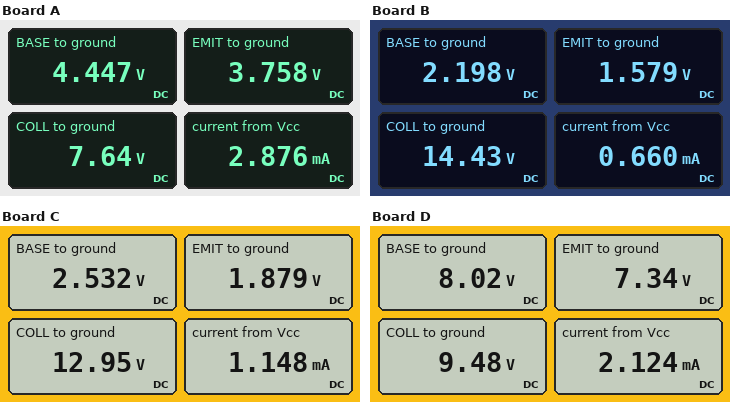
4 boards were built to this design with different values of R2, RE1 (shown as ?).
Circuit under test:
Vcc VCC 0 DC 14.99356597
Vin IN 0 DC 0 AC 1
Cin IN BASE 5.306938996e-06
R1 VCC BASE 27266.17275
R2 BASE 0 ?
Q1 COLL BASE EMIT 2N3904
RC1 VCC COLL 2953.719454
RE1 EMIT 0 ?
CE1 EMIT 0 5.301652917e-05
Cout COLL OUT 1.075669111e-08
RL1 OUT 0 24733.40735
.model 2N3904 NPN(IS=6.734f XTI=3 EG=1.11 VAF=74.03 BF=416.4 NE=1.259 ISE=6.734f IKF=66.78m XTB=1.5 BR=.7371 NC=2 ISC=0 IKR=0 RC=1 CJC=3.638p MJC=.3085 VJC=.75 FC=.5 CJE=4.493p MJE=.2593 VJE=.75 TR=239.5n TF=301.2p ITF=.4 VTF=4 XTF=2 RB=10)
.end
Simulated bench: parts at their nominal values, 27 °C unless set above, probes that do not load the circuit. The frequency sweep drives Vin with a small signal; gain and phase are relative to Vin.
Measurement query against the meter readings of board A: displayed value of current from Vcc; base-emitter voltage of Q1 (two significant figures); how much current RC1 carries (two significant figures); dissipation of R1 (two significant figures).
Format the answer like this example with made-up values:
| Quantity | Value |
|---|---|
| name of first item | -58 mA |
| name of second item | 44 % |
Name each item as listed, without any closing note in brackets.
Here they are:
| Quantity | Value |
|---|---|
| displayed value of current from Vcc | 2.876 mA |
| base-emitter voltage of Q1 | 690 mV |
| how much current RC1 carries | 2.5 mA |
| dissipation of R1 | 4.1 mW |
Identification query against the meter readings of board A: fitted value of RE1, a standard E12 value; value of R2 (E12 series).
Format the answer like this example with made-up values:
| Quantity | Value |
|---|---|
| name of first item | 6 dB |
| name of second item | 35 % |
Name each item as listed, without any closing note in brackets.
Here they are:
| Quantity | Value |
|---|---|
| fitted value of RE1, a standard E12 value | 1.5 kΩ |
| value of R2 | 12 kΩ |
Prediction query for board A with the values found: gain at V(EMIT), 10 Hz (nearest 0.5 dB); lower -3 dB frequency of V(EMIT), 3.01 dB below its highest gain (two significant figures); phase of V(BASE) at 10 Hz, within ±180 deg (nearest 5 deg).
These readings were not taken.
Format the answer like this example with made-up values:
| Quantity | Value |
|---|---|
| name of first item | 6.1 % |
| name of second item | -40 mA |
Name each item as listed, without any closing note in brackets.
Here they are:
| Quantity | Value |
|---|---|
| gain at V(EMIT), 10 Hz | -1.0 dB |
| lower -3 dB frequency of V(EMIT), 3.01 dB below its highest gain | 3.4 Hz |
| phase of V(BASE) at 10 Hz, within ±180 deg | 20 deg |
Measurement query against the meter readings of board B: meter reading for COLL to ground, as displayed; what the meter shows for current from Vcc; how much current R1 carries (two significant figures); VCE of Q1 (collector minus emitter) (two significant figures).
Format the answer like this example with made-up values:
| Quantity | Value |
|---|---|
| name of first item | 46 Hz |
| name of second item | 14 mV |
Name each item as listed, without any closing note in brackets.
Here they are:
| Quantity | Value |
|---|---|
| meter reading for COLL to ground, as displayed | 14.43 V |
| what the meter shows for current from Vcc | 0.660 mA |
| how much current R1 carries | 470 µA |
| VCE of Q1 (collector minus emitter) | 13 V |
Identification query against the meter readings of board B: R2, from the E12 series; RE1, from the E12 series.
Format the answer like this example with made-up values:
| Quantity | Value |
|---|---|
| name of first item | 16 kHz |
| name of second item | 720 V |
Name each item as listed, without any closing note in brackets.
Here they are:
| Quantity | Value |
|---|---|
| R2, from the E12 series | 4.7 kΩ |
| RE1, from the E12 series | 8.2 kΩ |
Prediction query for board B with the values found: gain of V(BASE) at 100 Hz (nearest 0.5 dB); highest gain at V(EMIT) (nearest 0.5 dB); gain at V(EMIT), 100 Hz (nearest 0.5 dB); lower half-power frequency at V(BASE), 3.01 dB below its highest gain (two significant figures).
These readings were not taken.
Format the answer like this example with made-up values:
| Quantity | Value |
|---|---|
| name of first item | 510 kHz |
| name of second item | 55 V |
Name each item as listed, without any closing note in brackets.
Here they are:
| Quantity | Value |
|---|---|
| gain of V(BASE) at 100 Hz | 0 dB |
| highest gain at V(EMIT) | -3.0 dB |
| gain at V(EMIT), 100 Hz | -13.5 dB |
| lower half-power frequency at V(BASE), 3.01 dB below its highest gain | 8.2 Hz |
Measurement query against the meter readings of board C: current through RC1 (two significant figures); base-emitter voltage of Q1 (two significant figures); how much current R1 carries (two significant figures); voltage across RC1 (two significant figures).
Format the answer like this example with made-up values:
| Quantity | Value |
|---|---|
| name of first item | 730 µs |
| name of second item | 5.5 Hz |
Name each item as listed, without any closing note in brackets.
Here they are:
| Quantity | Value |
|---|---|
| current through RC1 | 690 µA |
| base-emitter voltage of Q1 | 650 mV |
| how much current R1 carries | 460 µA |
| voltage across RC1 | 2.0 V |
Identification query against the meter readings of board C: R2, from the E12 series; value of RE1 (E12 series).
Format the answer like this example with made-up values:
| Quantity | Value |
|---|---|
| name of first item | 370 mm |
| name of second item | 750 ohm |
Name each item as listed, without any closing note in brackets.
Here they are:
| Quantity | Value |
|---|---|
| R2, from the E12 series | 5.6 kΩ |
| value of RE1 | 2.7 kΩ |
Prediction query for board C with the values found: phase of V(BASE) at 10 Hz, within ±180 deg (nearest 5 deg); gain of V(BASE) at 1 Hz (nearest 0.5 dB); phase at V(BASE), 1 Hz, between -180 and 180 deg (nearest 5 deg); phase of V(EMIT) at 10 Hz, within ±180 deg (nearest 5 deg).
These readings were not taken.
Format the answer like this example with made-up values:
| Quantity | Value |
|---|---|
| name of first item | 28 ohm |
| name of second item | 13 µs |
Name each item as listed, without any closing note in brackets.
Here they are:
| Quantity | Value |
|---|---|
| phase of V(BASE) at 10 Hz, within ±180 deg | 30 deg |
| gain of V(BASE) at 1 Hz | -16.5 dB |
| phase at V(BASE), 1 Hz, between -180 and 180 deg | 80 deg |
| phase of V(EMIT) at 10 Hz, within ±180 deg | 25 deg |
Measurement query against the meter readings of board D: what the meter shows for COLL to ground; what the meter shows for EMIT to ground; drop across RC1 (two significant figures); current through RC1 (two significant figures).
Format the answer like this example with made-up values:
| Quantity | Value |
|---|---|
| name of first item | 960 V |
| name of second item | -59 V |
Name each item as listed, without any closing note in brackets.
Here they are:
| Quantity | Value |
|---|---|
| what the meter shows for COLL to ground | 9.48 V |
| what the meter shows for EMIT to ground | 7.34 V |
| drop across RC1 | 5.5 V |
| current through RC1 | 1.9 mA |
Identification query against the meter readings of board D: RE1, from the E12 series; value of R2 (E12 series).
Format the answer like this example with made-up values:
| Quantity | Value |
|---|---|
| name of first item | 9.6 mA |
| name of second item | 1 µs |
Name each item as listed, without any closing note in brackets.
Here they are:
| Quantity | Value |
|---|---|
| RE1, from the E12 series | 3.9 kΩ |
| value of R2 | 33 kΩ |
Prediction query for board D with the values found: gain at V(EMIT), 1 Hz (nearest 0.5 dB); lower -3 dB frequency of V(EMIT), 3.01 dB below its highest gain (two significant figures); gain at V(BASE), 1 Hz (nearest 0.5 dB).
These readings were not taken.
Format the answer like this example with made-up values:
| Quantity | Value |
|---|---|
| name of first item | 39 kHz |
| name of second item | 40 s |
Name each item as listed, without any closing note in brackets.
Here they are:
| Quantity | Value |
|---|---|
| gain at V(EMIT), 1 Hz | -7.5 dB |
| lower -3 dB frequency of V(EMIT), 3.01 dB below its highest gain | 1.9 Hz |
| gain at V(BASE), 1 Hz | -7.5 dB |
